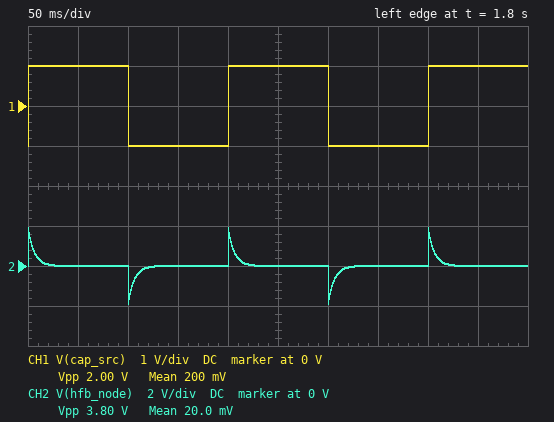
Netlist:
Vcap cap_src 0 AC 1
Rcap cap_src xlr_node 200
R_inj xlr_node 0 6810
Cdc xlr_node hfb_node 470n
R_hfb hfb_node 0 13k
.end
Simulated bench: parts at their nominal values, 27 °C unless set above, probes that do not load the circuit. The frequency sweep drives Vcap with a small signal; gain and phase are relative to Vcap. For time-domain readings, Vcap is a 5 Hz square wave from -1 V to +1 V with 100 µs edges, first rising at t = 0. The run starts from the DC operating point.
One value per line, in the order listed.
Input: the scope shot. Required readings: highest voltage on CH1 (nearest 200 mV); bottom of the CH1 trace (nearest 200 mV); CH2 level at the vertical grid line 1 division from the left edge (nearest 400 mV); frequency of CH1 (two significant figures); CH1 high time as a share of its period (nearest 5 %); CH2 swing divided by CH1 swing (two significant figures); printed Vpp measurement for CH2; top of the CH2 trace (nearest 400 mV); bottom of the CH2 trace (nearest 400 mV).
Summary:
1.0 V
-1.0 V
0 V
5.0 Hz
50 %
1.9
3.80 V
2.0 V
-2.0 V
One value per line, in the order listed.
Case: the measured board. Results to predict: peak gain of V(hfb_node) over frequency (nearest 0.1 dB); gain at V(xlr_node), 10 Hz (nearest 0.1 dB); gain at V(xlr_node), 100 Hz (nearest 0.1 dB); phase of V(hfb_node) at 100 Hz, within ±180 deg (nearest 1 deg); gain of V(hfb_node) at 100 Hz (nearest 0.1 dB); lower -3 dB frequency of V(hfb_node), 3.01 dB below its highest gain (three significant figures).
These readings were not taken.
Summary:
-0.4 dB
-0.3 dB
-0.4 dB
14 deg
-0.7 dB
25.7 Hz
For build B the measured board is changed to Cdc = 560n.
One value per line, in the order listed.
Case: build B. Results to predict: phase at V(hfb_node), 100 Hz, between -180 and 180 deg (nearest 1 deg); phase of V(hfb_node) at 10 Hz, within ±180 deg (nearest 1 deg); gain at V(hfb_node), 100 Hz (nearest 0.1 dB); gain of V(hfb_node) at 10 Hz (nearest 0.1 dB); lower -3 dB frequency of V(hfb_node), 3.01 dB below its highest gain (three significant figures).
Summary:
12 deg
65 deg
-0.6 dB
-7.9 dB
21.5 Hz
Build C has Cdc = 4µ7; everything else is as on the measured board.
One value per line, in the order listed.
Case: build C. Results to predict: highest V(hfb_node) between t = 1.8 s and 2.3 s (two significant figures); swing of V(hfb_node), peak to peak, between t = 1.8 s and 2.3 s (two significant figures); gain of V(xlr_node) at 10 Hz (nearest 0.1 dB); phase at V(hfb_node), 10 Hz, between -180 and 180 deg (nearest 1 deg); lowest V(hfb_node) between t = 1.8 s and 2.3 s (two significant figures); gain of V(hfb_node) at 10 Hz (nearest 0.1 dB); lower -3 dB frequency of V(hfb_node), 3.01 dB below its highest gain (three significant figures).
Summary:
1.6 V
3.2 V
-0.4 dB
14 deg
-1.6 V
-0.7 dB
2.57 Hz
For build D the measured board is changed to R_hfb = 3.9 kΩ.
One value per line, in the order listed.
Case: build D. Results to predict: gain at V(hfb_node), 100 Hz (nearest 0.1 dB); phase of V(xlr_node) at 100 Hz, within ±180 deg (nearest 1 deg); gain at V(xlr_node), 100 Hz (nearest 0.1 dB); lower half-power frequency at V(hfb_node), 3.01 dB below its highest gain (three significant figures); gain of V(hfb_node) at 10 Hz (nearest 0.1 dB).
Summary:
-2.9 dB
-1 deg
-0.5 dB
82.7 Hz
-19.1 dB
